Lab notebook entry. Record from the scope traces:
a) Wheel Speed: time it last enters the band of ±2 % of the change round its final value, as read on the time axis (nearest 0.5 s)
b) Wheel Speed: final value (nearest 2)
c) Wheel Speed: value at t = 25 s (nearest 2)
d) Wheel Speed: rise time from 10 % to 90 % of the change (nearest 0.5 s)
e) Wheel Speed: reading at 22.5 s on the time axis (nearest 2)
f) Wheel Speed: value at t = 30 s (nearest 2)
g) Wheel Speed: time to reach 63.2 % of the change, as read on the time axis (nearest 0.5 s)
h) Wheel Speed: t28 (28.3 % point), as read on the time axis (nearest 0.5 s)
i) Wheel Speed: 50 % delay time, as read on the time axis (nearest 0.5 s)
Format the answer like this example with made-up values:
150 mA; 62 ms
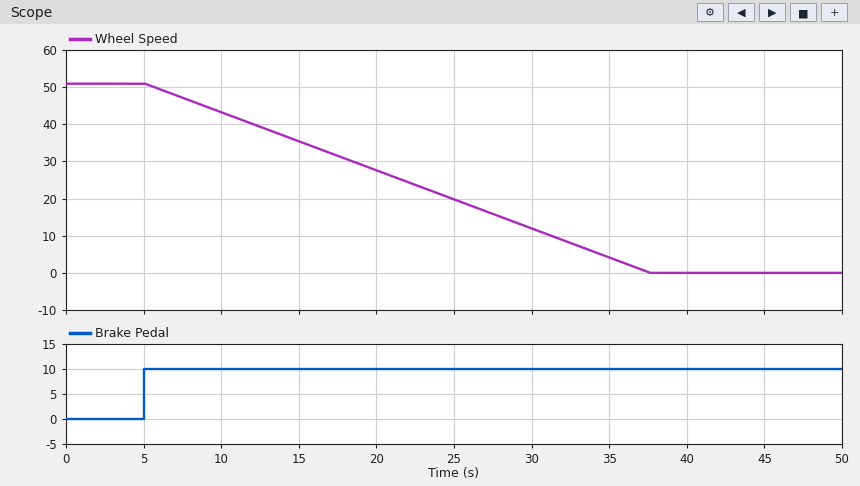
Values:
37.0 s; 0; 20; 26.0 s; 24; 12; 25.5 s; 14.5 s; 21.5 s
